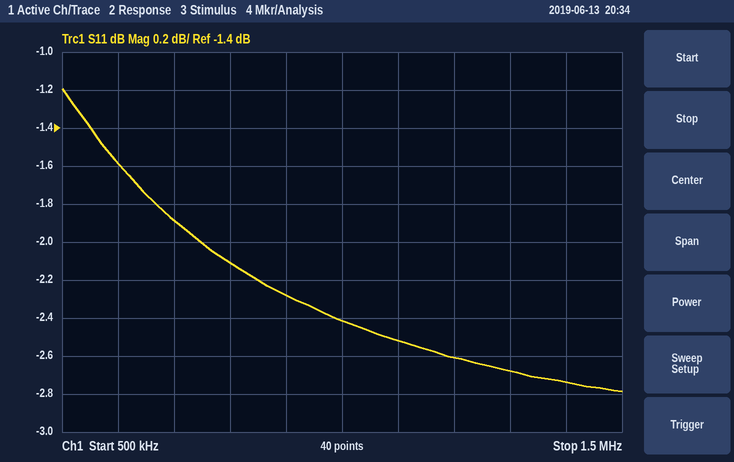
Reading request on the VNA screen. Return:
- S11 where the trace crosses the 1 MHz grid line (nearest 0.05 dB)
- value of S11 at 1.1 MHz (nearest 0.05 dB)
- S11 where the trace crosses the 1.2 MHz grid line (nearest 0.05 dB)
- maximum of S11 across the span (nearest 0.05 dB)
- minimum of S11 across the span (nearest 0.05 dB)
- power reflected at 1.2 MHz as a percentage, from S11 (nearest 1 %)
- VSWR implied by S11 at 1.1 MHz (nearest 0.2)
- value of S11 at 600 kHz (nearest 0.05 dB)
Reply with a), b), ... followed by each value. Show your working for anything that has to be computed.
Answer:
a) -2.40 dB
b) -2.50 dB
c) -2.60 dB
d) -1.20 dB
e) -2.80 dB
f) 10^(-2.6/10) ≈ 55 %
g) |Γ| = 10^(-2.5/20) = 0.7499; VSWR = (1 + 0.7499)/(1 − 0.7499) ≈ 7.0
h) -1.60 dB
